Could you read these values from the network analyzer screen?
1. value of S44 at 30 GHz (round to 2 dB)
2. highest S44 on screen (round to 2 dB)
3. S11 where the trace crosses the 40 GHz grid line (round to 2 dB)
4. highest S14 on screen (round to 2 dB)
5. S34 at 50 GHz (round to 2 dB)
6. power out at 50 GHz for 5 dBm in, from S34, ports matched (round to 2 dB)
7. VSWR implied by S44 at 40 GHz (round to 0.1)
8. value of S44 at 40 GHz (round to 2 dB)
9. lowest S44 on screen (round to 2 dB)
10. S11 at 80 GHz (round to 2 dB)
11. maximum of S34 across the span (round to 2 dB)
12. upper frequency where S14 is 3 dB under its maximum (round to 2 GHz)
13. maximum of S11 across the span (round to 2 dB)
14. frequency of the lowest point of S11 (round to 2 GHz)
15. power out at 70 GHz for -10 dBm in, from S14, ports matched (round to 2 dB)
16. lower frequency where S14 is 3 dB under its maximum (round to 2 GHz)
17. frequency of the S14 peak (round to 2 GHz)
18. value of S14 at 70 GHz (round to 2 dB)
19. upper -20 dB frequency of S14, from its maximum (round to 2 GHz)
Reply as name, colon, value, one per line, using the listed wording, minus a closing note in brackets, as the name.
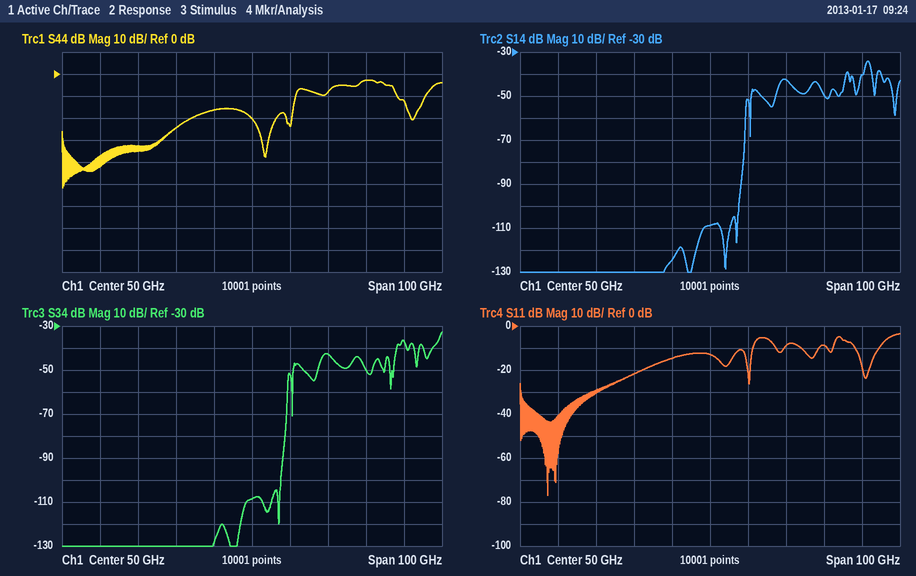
value of S44 at 30 GHz: -24 dB
highest S44 on screen: -2 dB
S11 where the trace crosses the 40 GHz grid line: -14 dB
highest S14 on screen: -34 dB
S34 at 50 GHz: -108 dB
power out at 50 GHz for 5 dBm in, from S34, ports matched: -104 dBm
VSWR implied by S44 at 40 GHz: 1.4
value of S44 at 40 GHz: -16 dB
lowest S44 on screen: -52 dB
S11 at 80 GHz: -8 dB
maximum of S34 across the span: -32 dB
upper frequency where S14 is 3 dB under its maximum: 92 GHz
maximum of S11 across the span: -4 dB
frequency of the lowest point of S11: 8 GHz
power out at 70 GHz for -10 dBm in, from S14, ports matched: -52 dBm
lower frequency where S14 is 3 dB under its maximum: 90 GHz
frequency of the S14 peak: 92 GHz
value of S14 at 70 GHz: -42 dB
upper -20 dB frequency of S14, from its maximum: 98 GHz
